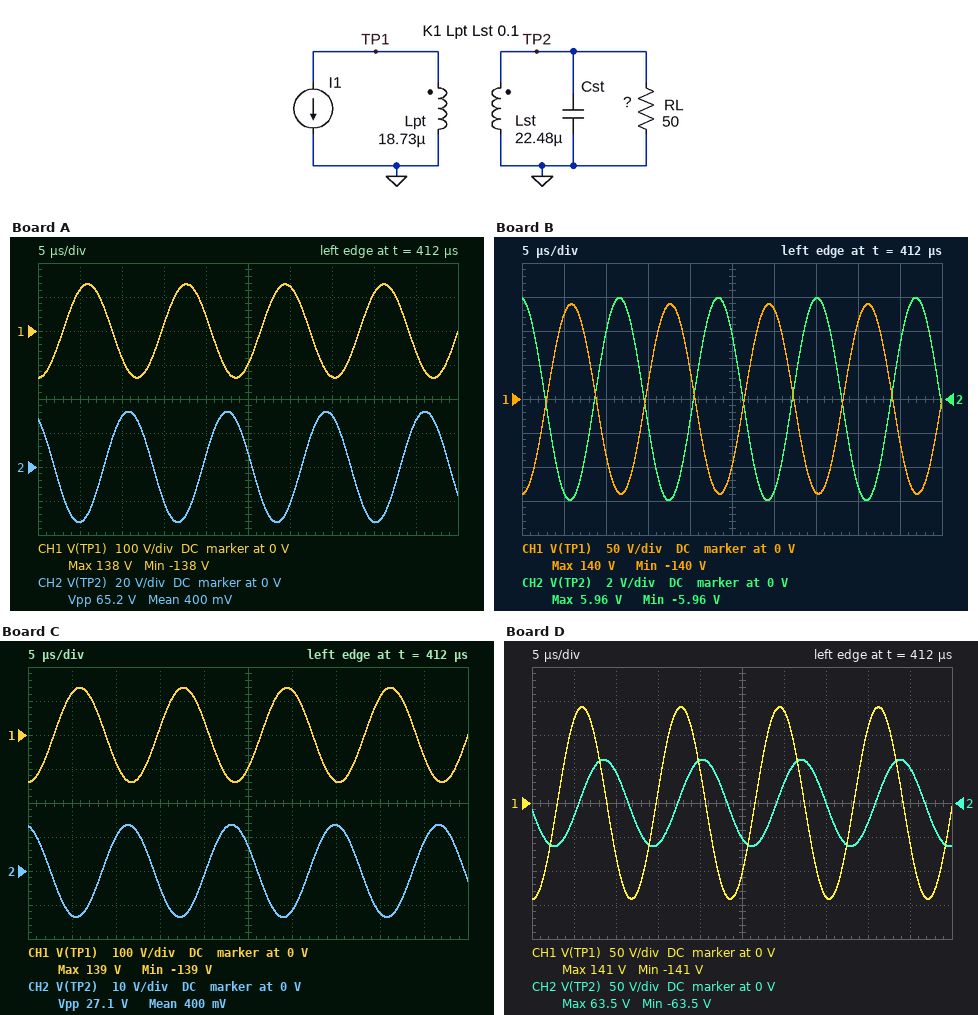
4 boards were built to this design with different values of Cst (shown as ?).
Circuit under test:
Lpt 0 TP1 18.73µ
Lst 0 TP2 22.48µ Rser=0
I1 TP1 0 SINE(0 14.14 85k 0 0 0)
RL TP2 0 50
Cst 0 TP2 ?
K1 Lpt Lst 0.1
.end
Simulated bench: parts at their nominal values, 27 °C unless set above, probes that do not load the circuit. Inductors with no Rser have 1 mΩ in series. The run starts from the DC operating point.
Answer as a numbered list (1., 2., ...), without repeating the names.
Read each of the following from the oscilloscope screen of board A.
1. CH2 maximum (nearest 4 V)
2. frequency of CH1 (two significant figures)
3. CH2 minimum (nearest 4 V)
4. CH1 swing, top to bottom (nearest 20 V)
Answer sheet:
1. 32 V
2. 85 kHz
3. -32 V
4. 280 V
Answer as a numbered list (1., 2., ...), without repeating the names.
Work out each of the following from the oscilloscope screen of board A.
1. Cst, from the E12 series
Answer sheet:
1. 220 nF
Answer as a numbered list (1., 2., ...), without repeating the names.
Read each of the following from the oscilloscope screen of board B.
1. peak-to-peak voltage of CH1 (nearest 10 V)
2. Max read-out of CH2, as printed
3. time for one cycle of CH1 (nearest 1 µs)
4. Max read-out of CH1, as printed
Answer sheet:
1. 280 V
2. 5.96 V
3. 12 µs
4. 140 V
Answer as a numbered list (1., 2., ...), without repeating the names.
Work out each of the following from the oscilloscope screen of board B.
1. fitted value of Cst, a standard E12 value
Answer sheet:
1. 560 nF
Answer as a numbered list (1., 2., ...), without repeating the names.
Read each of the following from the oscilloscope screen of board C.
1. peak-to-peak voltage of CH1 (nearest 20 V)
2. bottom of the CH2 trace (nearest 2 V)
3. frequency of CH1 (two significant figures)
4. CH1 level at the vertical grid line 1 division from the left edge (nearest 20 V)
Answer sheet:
1. 280 V
2. -14 V
3. 85 kHz
4. 120 V
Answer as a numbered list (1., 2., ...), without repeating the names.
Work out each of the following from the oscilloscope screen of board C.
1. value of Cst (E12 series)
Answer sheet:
1. 330 nF
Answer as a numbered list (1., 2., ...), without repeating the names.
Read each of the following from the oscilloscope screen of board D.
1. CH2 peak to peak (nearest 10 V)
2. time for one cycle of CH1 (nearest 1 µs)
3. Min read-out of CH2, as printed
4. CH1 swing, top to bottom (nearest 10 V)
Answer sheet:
1. 130 V
2. 12 µs
3. -63.5 V
4. 280 V
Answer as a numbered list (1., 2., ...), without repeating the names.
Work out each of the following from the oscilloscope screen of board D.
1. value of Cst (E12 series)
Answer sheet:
1. 150 nF
